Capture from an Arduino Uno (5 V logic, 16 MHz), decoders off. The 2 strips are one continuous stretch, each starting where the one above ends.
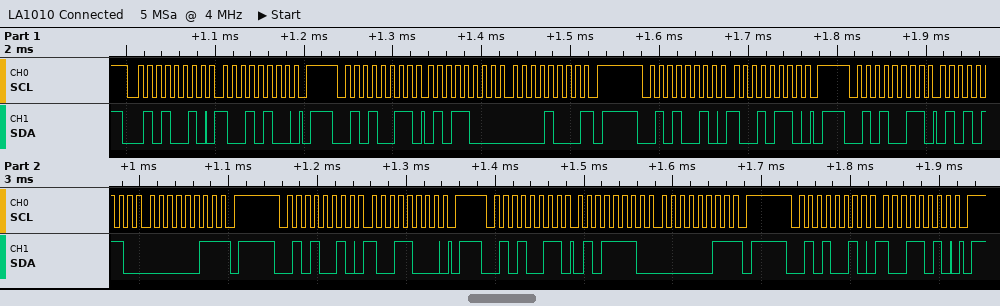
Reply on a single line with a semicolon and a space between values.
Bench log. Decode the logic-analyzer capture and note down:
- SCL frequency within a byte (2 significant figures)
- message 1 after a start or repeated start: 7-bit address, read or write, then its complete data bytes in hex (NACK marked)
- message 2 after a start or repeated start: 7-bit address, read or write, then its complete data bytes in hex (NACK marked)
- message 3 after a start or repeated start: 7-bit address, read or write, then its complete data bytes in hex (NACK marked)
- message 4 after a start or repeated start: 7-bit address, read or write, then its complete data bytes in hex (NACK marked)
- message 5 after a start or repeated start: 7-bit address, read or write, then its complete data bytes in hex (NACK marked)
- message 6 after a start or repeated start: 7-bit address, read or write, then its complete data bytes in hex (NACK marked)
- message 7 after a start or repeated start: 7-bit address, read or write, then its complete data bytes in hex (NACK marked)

100 kHz; 0x29 write: 94; 0x29 read: 58 08 NACK; 0x29 write: 96; 0x29 read: 56 03 NACK; 0x29 write: 98; 0x29 read: 5E 03 NACK; 0x29 write: 9A
